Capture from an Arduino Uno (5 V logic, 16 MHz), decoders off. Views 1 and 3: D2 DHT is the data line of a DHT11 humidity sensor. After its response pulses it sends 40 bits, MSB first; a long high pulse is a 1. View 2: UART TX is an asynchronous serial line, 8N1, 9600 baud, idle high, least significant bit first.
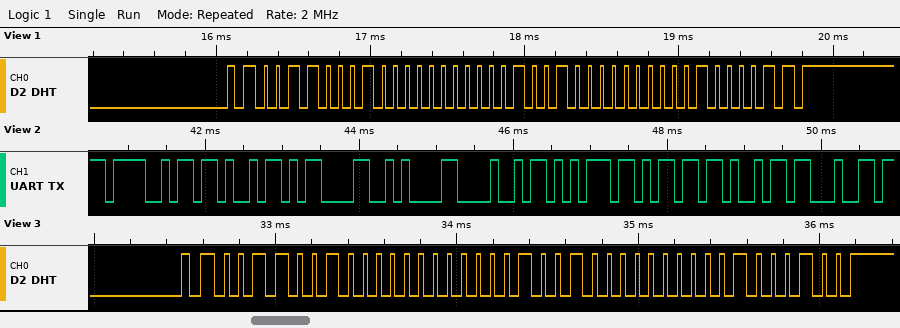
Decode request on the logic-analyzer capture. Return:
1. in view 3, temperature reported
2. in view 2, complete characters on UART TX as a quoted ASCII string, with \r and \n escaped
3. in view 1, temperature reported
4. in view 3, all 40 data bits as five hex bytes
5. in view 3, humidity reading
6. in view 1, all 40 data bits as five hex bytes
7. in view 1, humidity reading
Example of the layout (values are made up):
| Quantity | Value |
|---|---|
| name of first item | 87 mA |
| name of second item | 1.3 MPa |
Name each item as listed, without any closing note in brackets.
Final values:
| Quantity | Value |
|---|---|
| in view 3, temperature reported | 18.0 °C |
| in view 2, complete characters on UART TX as a quoted ASCII string, with \r and \n escaped | "OK\r\nHumid" |
| in view 1, temperature reported | 18.0 °C |
| in view 3, all 40 data bits as five hex bytes | 32 00 12 00 44 |
| in view 3, humidity reading | 50 % |
| in view 1, all 40 data bits as five hex bytes | 31 00 12 00 43 |
| in view 1, humidity reading | 49 % |
